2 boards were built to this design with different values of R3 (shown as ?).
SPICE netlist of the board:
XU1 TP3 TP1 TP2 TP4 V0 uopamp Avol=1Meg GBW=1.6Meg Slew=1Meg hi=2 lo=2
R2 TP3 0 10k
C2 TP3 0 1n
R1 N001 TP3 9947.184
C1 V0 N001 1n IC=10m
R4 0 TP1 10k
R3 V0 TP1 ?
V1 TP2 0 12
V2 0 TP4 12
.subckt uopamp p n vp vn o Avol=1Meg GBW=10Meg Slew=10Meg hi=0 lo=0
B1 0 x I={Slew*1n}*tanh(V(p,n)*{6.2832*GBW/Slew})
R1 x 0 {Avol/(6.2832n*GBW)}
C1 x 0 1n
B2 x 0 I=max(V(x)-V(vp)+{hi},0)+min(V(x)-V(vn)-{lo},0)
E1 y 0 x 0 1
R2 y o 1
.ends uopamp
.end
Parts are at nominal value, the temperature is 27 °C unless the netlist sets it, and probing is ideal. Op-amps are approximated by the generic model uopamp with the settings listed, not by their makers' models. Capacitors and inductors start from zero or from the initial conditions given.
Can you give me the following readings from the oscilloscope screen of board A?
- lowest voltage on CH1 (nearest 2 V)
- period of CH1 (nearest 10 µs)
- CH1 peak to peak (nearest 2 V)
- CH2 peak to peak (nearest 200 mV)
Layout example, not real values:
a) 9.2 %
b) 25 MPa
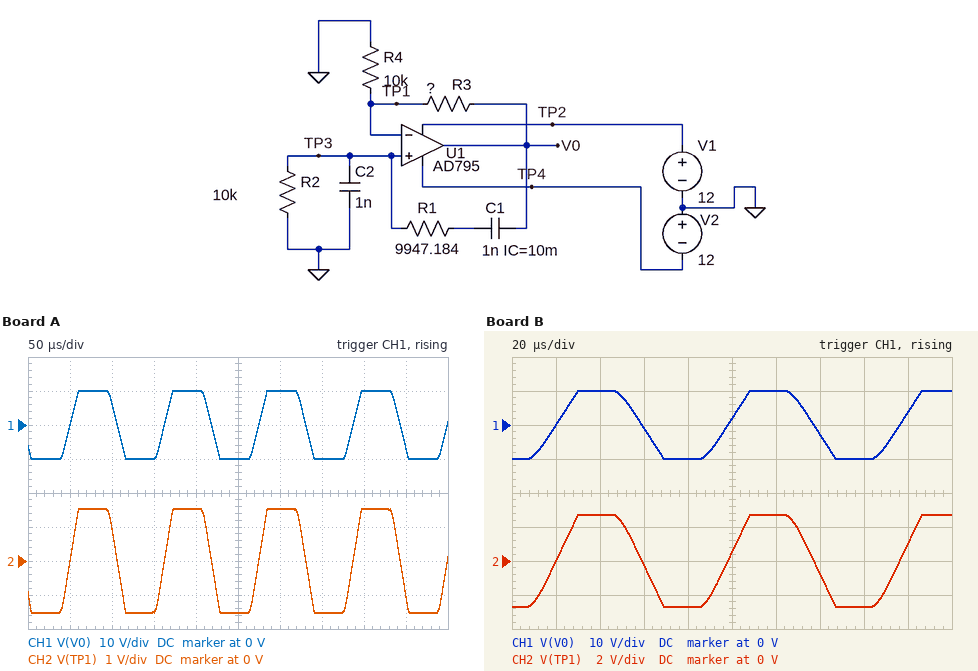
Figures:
a) -10 V
b) 110 µs
c) 20 V
d) 3.0 V
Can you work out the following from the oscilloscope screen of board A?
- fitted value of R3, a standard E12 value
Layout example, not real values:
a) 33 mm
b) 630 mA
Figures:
a) 56 kΩ
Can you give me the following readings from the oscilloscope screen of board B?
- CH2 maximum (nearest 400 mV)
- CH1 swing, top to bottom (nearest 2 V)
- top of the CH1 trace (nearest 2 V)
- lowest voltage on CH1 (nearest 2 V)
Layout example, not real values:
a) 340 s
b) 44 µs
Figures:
a) 2.8 V
b) 20 V
c) 10 V
d) -10 V
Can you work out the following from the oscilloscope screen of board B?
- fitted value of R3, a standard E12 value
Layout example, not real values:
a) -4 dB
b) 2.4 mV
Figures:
a) 27 kΩ
